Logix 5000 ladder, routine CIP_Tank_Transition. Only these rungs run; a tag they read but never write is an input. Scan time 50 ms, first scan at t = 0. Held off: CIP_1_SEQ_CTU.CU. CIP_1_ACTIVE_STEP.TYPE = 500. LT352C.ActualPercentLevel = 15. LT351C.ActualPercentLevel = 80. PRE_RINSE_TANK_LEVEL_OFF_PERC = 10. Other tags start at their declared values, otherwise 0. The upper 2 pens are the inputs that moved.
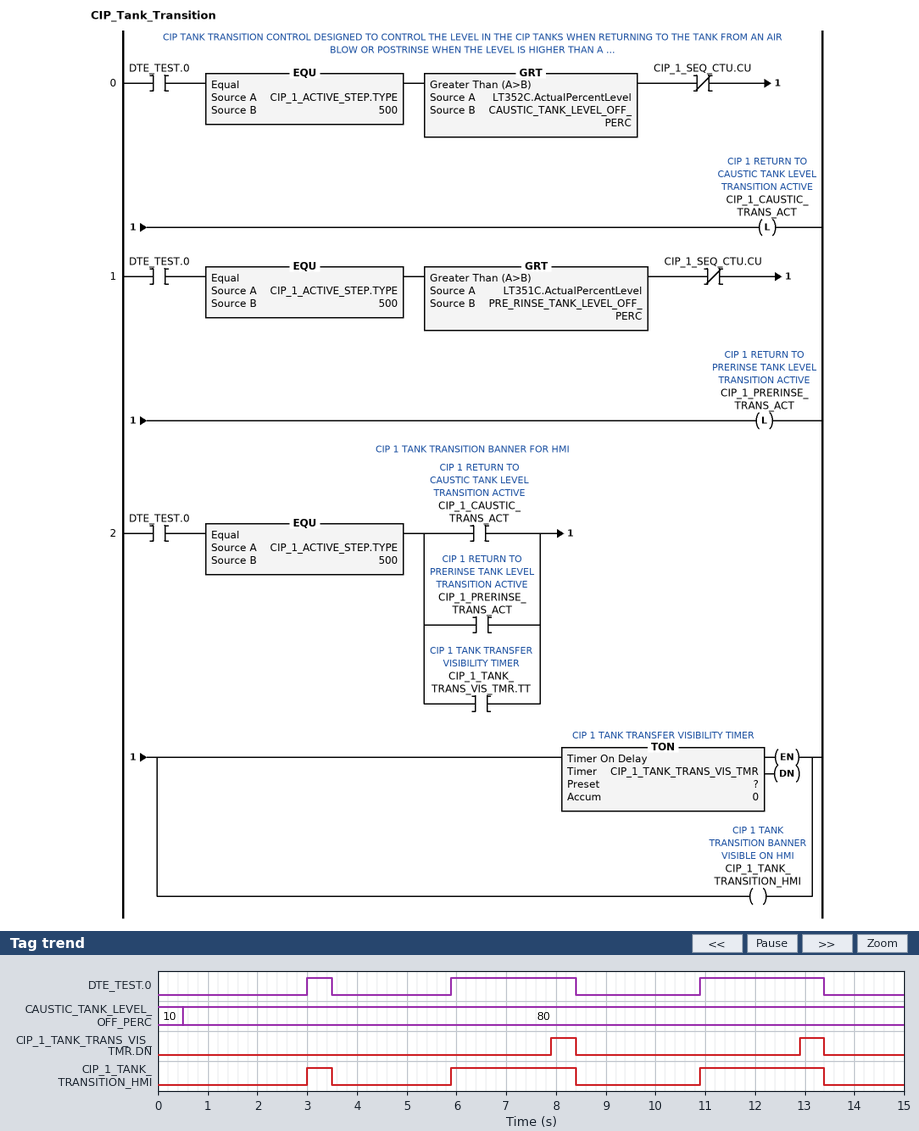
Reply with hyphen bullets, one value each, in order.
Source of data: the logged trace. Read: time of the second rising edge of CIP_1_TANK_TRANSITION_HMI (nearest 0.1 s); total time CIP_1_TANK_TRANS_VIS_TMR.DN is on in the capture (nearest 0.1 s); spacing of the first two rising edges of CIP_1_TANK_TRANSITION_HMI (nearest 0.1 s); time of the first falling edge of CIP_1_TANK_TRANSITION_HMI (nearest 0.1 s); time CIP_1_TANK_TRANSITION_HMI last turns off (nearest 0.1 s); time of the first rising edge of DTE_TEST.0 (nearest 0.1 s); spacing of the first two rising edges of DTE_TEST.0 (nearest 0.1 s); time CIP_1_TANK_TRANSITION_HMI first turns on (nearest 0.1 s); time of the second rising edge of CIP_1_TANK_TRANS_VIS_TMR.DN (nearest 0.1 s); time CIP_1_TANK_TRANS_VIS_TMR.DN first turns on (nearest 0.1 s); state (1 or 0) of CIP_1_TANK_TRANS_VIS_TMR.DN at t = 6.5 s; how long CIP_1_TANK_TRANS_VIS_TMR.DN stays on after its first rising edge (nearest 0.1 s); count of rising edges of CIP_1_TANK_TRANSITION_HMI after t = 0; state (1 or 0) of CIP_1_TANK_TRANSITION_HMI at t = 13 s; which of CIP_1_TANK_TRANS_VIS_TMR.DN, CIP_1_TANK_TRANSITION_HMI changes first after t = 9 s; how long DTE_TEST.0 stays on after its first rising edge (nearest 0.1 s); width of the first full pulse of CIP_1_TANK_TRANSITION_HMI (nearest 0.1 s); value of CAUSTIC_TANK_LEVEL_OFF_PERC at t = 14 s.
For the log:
- 5.9 s
- 1.0 s
- 2.9 s
- 3.5 s
- 13.4 s
- 3.0 s
- 2.9 s
- 3.0 s
- 12.9 s
- 7.9 s
- 0
- 0.5 s
- 3
- 1
- CIP_1_TANK_TRANSITION_HMI
- 0.5 s
- 0.5 s
- 80
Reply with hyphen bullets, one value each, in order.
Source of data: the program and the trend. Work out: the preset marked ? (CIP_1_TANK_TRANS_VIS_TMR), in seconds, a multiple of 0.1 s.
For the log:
- 2.0 s
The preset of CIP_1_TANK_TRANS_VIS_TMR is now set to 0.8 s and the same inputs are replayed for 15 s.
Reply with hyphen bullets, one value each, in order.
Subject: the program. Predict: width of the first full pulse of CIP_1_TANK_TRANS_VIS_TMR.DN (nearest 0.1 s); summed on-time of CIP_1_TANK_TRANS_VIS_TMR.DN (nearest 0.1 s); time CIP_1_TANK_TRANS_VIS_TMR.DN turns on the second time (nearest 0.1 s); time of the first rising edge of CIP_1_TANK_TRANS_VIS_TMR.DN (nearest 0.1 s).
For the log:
- 1.7 s
- 3.4 s
- 11.7 s
- 6.7 s
